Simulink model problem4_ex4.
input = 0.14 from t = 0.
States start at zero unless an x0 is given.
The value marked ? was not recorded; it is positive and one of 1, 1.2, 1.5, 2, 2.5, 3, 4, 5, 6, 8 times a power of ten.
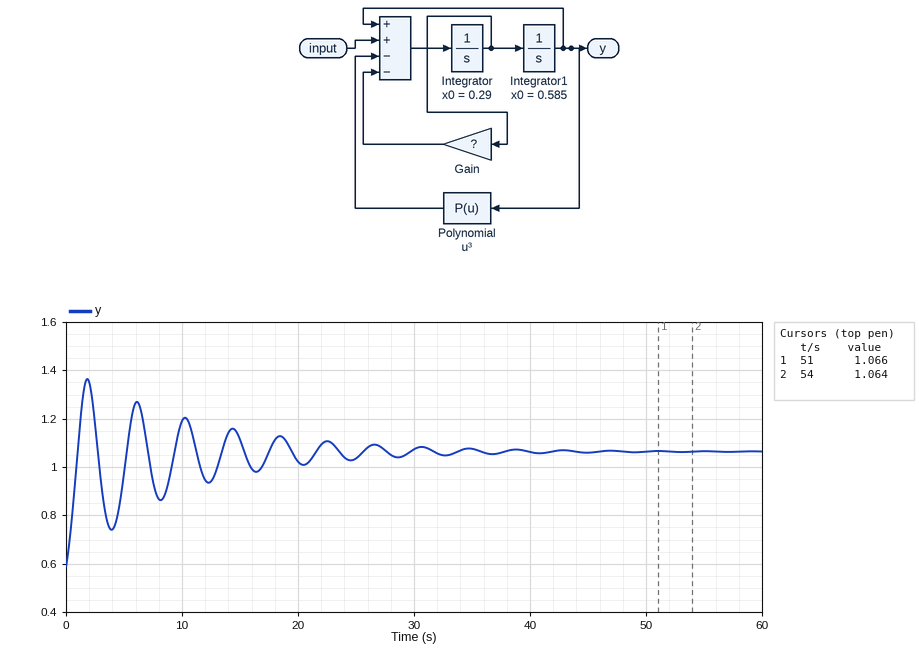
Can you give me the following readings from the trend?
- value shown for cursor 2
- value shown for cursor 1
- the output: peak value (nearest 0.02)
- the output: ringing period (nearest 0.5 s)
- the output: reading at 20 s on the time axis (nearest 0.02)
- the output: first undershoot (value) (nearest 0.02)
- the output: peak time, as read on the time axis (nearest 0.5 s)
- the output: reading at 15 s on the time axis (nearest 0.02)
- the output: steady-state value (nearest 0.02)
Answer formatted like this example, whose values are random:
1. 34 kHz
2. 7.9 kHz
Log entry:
1. 1.064
2. 1.066
3. 1.36
4. 4.5 s
5. 1.02
6. 0.74
7. 2.0 s
8. 1.12
9. 1.06
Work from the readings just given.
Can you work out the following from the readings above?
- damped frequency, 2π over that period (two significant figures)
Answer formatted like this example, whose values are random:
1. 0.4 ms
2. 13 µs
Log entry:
1. 1.4 rad/s
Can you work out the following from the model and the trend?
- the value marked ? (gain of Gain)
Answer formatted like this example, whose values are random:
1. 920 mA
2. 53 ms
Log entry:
1. 0.2
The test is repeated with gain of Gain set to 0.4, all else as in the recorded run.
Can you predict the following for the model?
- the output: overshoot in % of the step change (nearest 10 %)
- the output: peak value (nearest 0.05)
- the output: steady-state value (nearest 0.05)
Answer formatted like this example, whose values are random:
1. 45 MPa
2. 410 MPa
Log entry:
1. 50 %
2. 1.30
3. 1.05
